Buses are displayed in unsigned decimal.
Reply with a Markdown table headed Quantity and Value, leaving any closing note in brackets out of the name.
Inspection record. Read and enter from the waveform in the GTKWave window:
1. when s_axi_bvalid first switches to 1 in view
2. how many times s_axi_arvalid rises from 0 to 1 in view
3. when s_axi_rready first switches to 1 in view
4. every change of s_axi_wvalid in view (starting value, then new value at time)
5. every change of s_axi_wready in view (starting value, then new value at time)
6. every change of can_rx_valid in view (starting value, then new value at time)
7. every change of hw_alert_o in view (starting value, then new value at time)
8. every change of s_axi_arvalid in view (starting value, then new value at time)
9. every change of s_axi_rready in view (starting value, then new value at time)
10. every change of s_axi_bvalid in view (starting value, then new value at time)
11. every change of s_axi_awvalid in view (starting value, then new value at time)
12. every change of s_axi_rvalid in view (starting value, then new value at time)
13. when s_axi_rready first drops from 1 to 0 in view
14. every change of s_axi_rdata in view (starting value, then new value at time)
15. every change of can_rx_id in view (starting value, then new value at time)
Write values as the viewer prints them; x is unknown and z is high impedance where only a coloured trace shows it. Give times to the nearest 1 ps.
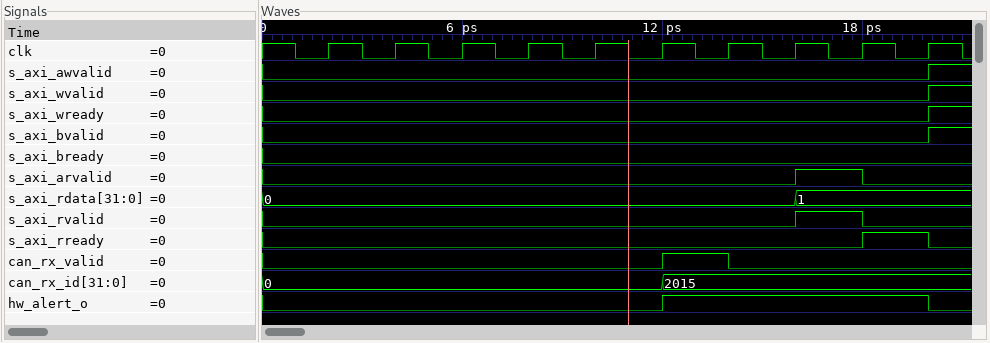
| Quantity | Value |
|---|---|
| when s_axi_bvalid first switches to 1 in view | 20 ps |
| how many times s_axi_arvalid rises from 0 to 1 in view | 1 |
| when s_axi_rready first switches to 1 in view | 18 ps |
| every change of s_axi_wvalid in view | 0, 1 at 20 ps |
| every change of s_axi_wready in view | 0, 1 at 20 ps |
| every change of can_rx_valid in view | 0, 1 at 12 ps, 0 at 14 ps |
| every change of hw_alert_o in view | 0, 1 at 12 ps, 0 at 20 ps |
| every change of s_axi_arvalid in view | 0, 1 at 16 ps, 0 at 18 ps |
| every change of s_axi_rready in view | 0, 1 at 18 ps, 0 at 20 ps |
| every change of s_axi_bvalid in view | 0, 1 at 20 ps |
| every change of s_axi_awvalid in view | 0, 1 at 20 ps |
| every change of s_axi_rvalid in view | 0, 1 at 16 ps, 0 at 18 ps |
| when s_axi_rready first drops from 1 to 0 in view | 20 ps |
| every change of s_axi_rdata in view | 0, 1 at 16 ps |
| every change of can_rx_id in view | 0, 2015 at 12 ps |
